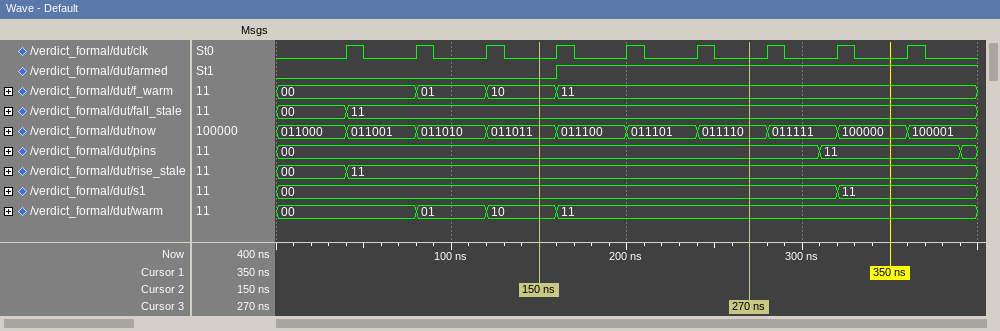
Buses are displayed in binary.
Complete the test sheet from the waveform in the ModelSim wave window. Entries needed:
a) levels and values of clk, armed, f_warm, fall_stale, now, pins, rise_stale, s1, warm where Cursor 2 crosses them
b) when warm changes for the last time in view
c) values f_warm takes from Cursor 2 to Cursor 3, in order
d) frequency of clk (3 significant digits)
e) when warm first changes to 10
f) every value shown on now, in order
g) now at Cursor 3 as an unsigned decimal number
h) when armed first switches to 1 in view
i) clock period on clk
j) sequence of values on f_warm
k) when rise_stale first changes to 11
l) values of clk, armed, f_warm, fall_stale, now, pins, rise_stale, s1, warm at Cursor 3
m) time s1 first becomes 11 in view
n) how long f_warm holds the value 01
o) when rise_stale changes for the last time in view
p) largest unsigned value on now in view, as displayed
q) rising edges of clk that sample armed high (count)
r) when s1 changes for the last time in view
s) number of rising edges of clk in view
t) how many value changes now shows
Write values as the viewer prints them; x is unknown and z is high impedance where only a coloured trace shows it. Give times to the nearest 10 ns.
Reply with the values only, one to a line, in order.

clk=0, armed=0, f_warm=10, fall_stale=11, now=011011, pins=00, rise_stale=11, s1=00, warm=10
160 ns
10, 11
25.0 MHz
120 ns
011000, 011001, 011010, 011011, 011100, 011101, 011110, 011111, 100000, 100001
30
160 ns
40 ns
00, 01, 10, 11
40 ns
clk=0, armed=1, f_warm=11, fall_stale=11, now=011110, pins=00, rise_stale=11, s1=00, warm=11
320 ns
40 ns
40 ns
100001
5
320 ns
9
9
